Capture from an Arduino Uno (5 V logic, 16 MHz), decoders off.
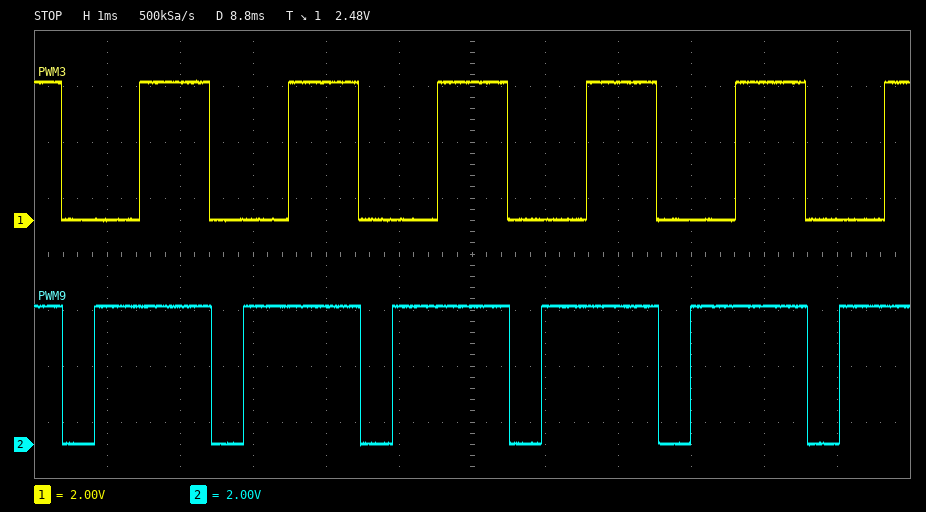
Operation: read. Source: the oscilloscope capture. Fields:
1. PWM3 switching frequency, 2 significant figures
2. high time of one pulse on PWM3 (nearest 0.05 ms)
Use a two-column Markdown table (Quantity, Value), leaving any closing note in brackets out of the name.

| Quantity | Value |
|---|---|
| PWM3 switching frequency, 2 significant figures | 490 Hz |
| high time of one pulse on PWM3 | 0.95 ms |
